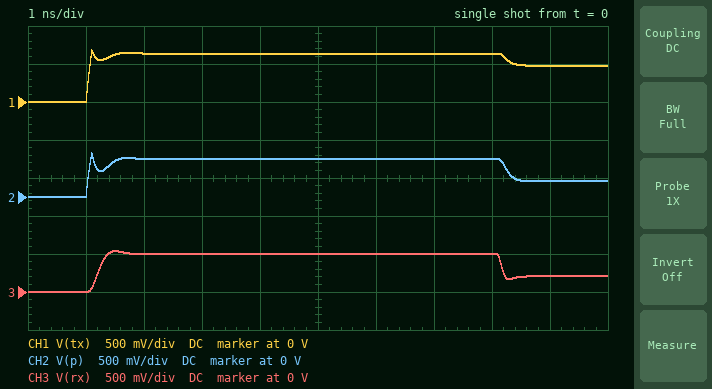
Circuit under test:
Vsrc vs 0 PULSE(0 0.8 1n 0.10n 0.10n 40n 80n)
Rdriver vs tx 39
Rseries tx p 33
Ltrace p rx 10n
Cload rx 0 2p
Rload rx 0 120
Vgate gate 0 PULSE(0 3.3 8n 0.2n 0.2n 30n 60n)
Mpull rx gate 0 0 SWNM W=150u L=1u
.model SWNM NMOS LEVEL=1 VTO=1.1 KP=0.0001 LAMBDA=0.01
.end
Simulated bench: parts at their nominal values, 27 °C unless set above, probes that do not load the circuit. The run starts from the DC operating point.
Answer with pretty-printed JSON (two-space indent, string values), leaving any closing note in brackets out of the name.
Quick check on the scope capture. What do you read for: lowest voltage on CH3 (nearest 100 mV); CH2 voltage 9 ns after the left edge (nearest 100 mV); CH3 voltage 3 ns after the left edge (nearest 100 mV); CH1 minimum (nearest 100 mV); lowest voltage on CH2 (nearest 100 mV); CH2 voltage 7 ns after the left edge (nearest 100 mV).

{
  "lowest voltage on CH3": "0 V",
  "CH2 voltage 9 ns after the left edge": "200 mV",
  "CH3 voltage 3 ns after the left edge": "500 mV",
  "CH1 minimum": "0 V",
  "lowest voltage on CH2": "0 V",
  "CH2 voltage 7 ns after the left edge": "500 mV"
}
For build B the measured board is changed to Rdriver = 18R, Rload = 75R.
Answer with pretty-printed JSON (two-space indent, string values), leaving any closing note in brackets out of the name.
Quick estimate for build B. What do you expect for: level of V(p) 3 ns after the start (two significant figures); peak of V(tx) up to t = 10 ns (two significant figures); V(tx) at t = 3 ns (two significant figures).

{
  "level of V(p) 3 ns after the start": "480 mV",
  "peak of V(tx) up to t = 10 ns": "740 mV",
  "V(tx) at t = 3 ns": "690 mV"
}
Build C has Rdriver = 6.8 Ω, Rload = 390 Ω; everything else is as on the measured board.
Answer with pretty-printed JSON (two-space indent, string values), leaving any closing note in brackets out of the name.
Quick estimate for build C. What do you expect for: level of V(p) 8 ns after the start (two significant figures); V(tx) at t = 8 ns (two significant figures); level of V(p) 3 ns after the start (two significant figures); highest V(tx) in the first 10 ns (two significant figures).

{
  "level of V(p) 8 ns after the start": "730 mV",
  "V(tx) at t = 8 ns": "790 mV",
  "level of V(p) 3 ns after the start": "720 mV",
  "highest V(tx) in the first 10 ns": "800 mV"
}
